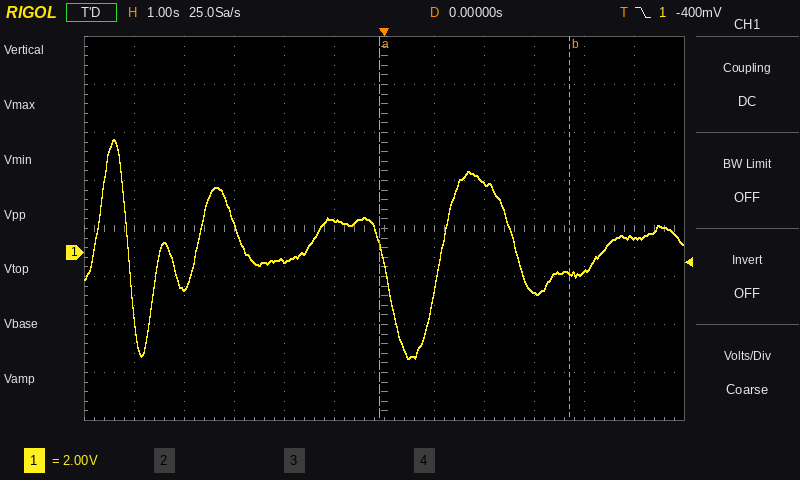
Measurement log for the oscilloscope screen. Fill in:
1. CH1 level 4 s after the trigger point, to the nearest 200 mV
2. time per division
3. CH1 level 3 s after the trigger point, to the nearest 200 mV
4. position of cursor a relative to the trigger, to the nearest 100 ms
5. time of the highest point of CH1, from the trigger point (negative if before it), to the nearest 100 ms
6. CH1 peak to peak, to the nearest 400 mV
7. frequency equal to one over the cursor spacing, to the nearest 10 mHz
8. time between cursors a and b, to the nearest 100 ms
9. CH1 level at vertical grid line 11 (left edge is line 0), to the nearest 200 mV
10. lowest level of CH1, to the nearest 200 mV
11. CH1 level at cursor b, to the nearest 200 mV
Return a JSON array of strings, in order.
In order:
["-800 mV", "1 s", "-1.6 V", "-100 ms", "-5.4 s", "9.2 V", "260 mHz", "3.8 s", "600 mV", "-4.4 V", "-800 mV"]
